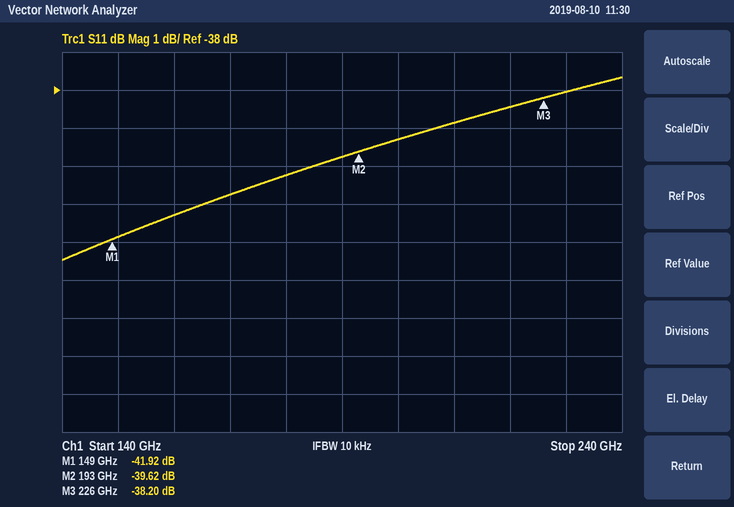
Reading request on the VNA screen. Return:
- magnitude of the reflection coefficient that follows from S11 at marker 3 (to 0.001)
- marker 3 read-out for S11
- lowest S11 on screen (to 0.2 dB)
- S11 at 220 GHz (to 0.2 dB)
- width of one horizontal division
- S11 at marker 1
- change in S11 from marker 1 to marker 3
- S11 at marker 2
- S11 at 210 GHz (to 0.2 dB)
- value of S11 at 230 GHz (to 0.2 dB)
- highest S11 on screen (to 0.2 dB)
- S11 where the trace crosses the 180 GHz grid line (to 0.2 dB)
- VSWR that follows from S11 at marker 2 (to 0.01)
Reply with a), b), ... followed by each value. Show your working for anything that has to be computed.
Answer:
a) 10^(-38.2/20) ≈ 0.012
b) -38.20 dB
c) -42.4 dB
d) -38.4 dB
e) 10 GHz
f) -41.92 dB
g) -38.2 − (-41.92) = 3.72 dB
h) -39.62 dB
i) -38.8 dB
j) -38.0 dB
k) -37.6 dB
l) -40.2 dB
m) (1 + 0.0104)/(1 − 0.0104) ≈ 1.02
